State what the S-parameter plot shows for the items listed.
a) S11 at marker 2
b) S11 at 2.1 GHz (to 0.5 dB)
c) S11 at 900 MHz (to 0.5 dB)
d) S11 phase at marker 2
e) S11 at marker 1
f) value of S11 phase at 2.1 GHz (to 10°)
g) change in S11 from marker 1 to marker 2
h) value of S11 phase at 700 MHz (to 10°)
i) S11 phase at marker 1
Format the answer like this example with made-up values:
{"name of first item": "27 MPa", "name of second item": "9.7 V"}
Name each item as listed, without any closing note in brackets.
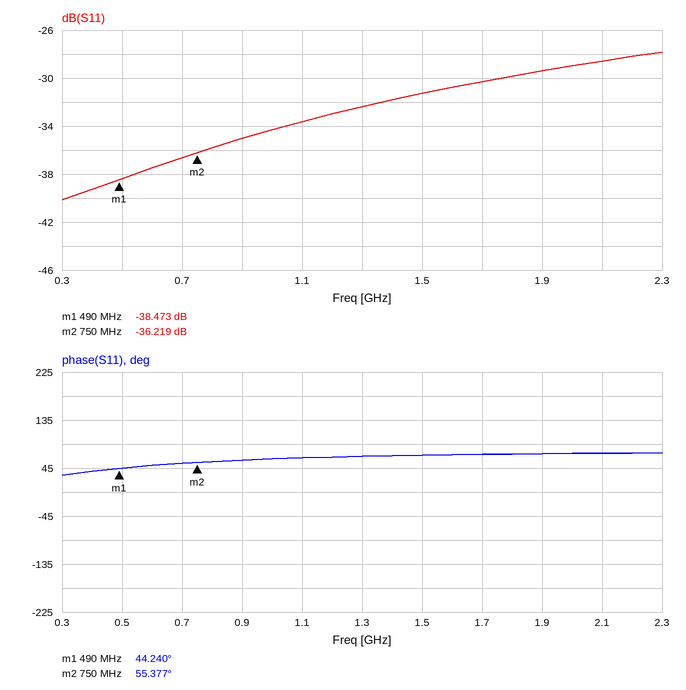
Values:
{"S11 at marker 2": "-36.219 dB", "S11 at 2.1 GHz": "-28.5 dB", "S11 at 900 MHz": "-35.0 dB", "S11 phase at marker 2": "55.377°", "S11 at marker 1": "-38.473 dB", "value of S11 phase at 2.1 GHz": "70°", "change in S11 from marker 1 to marker 2": "2.254 dB", "value of S11 phase at 700 MHz": "50°", "S11 phase at marker 1": "44.240°"}
